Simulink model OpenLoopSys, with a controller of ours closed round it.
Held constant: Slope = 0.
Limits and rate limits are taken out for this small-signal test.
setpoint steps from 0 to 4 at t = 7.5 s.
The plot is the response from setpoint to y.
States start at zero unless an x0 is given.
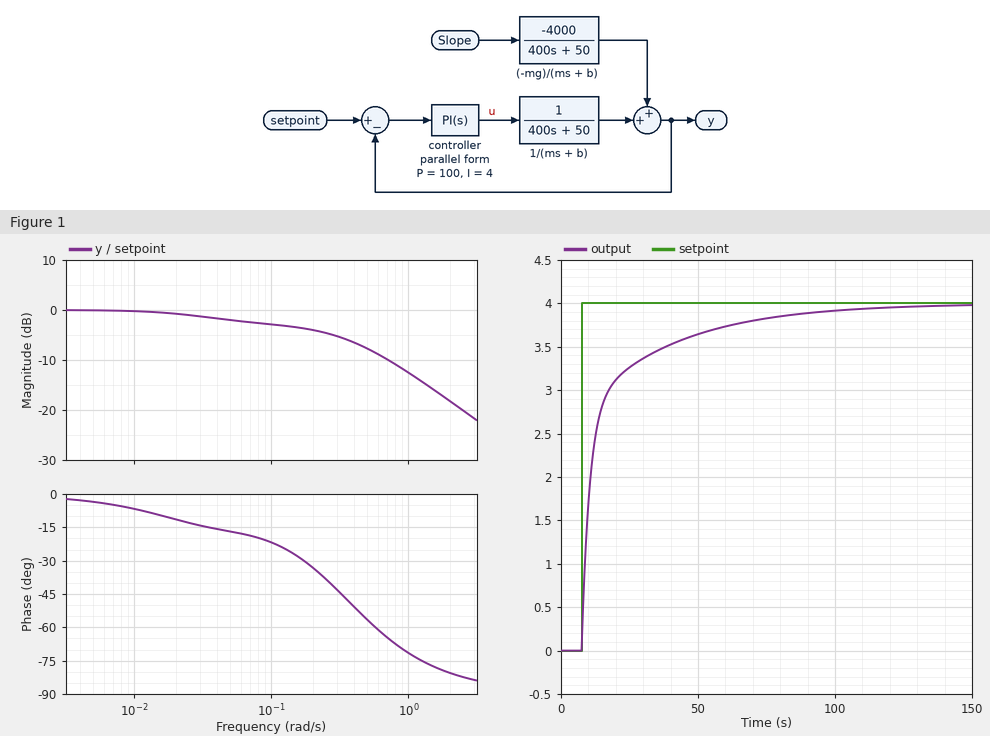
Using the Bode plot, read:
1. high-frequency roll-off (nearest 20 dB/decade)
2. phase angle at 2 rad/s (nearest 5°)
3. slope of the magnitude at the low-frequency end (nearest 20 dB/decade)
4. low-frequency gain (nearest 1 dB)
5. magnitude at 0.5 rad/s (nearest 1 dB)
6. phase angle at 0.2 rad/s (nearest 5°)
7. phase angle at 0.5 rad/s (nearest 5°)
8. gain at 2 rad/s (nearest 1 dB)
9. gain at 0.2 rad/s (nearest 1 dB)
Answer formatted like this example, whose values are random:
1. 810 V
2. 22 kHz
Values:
1. -20 dB/decade
2. -80°
3. 0 dB/decade
4. 0 dB
5. -8 dB
6. -35°
7. -55°
8. -18 dB
9. -4 dB
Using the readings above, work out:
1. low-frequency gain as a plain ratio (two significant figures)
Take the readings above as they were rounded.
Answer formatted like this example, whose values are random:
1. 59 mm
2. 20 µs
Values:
1. 1.0
